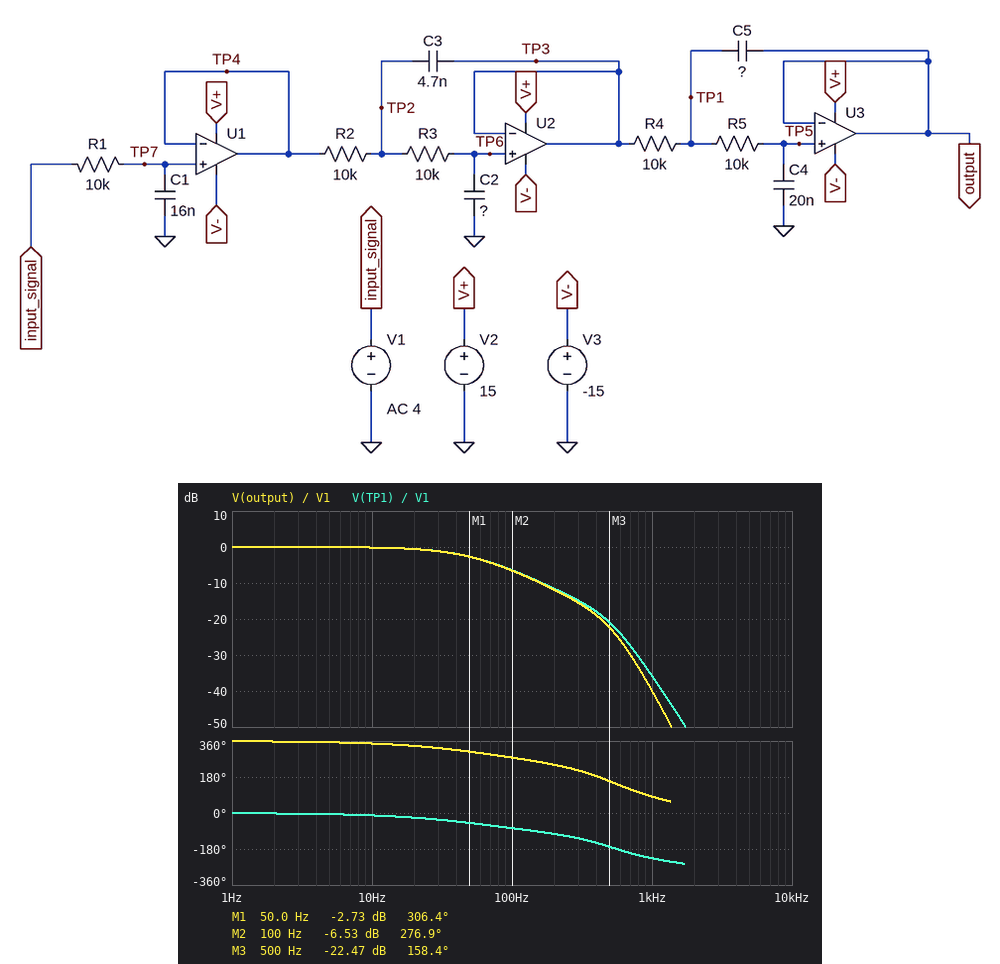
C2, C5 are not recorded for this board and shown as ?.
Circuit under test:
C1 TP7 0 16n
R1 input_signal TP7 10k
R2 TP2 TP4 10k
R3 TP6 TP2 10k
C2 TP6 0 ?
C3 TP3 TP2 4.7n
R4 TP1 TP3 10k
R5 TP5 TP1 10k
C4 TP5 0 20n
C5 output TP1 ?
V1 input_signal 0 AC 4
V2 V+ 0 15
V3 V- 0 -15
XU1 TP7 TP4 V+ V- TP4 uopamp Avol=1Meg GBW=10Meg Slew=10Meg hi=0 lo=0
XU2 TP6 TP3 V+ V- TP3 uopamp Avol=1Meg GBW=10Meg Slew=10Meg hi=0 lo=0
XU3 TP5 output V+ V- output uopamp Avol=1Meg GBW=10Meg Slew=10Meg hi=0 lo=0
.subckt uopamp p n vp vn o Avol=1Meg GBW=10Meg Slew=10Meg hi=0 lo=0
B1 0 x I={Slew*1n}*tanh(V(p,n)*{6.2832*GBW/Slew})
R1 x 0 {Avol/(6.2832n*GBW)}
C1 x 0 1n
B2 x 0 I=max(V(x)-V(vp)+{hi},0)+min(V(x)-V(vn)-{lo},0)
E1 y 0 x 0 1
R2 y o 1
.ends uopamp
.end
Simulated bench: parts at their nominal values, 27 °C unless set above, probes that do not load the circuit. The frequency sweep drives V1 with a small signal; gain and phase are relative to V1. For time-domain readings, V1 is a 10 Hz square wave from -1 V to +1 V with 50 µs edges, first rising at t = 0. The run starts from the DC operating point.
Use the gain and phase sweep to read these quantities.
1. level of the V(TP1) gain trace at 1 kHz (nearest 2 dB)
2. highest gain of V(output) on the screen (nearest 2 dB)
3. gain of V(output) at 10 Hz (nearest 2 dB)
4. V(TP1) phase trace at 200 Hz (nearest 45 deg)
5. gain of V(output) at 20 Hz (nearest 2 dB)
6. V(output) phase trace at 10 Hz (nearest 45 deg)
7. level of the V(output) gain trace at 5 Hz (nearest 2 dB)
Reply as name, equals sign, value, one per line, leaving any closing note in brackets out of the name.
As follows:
level of the V(TP1) gain trace at 1 kHz = -36 dB
highest gain of V(output) on the screen = 0 dB
gain of V(output) at 10 Hz = 0 dB
V(TP1) phase trace at 200 Hz = -90 deg
gain of V(output) at 20 Hz = 0 dB
V(output) phase trace at 10 Hz = 360 deg
level of the V(output) gain trace at 5 Hz = 0 dB
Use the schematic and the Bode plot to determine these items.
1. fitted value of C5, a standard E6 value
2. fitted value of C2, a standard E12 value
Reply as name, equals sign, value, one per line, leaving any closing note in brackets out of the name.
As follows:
fitted value of C5, a standard E6 value = 47 nF
fitted value of C2, a standard E12 value = 150 nF
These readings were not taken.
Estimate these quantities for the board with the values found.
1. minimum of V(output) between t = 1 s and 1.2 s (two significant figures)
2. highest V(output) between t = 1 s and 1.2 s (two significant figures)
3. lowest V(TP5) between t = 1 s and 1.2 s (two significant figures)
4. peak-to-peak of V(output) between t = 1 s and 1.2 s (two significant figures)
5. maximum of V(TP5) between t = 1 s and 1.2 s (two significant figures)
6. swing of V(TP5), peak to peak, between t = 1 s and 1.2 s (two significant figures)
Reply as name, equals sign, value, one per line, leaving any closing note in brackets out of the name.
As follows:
minimum of V(output) between t = 1 s and 1.2 s = -1.0 V
highest V(output) between t = 1 s and 1.2 s = 1.0 V
lowest V(TP5) between t = 1 s and 1.2 s = -1.0 V
peak-to-peak of V(output) between t = 1 s and 1.2 s = 2.0 V
maximum of V(TP5) between t = 1 s and 1.2 s = 1.0 V
swing of V(TP5), peak to peak, between t = 1 s and 1.2 s = 2.0 V
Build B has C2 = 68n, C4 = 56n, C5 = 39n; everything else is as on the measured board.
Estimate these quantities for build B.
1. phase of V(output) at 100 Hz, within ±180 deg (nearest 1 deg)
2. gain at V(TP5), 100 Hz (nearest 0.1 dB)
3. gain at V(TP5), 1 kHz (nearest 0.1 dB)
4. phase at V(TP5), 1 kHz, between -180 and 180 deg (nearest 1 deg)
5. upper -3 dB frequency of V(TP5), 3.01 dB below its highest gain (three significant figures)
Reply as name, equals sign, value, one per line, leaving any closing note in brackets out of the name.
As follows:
phase of V(output) at 100 Hz, within ±180 deg = -84 deg
gain at V(TP5), 100 Hz = -3.6 dB
gain at V(TP5), 1 kHz = -42.0 dB
phase at V(TP5), 1 kHz, between -180 and 180 deg = 86 deg
upper -3 dB frequency of V(TP5), 3.01 dB below its highest gain = 89.8 Hz
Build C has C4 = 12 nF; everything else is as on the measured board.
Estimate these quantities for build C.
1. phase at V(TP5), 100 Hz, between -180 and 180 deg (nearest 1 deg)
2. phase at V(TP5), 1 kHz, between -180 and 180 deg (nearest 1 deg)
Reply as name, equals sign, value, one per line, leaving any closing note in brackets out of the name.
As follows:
phase at V(TP5), 100 Hz, between -180 and 180 deg = -77 deg
phase at V(TP5), 1 kHz, between -180 and 180 deg = 90 deg
